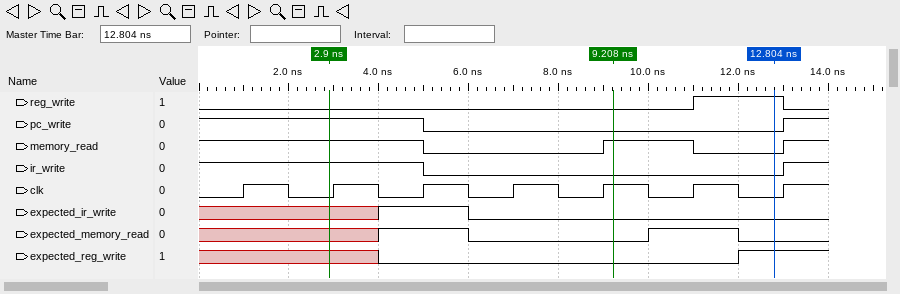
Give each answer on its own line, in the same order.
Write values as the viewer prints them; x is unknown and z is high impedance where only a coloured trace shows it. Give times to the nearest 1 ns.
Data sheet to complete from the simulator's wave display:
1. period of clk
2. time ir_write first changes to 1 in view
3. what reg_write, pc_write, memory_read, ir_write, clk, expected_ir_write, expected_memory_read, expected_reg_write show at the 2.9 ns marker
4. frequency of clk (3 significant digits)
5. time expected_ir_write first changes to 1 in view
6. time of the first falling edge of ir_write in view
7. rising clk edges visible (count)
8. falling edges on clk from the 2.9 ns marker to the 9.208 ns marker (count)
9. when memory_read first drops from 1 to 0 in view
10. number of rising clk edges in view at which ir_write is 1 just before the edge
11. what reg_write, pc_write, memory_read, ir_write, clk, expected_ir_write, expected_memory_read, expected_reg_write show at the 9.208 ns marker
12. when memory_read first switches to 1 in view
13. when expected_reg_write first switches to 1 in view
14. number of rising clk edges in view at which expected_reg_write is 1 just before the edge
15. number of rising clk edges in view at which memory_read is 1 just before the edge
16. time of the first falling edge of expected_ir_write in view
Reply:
2 ns
13 ns
reg_write=0, pc_write=1, memory_read=1, ir_write=1, clk=0, expected_ir_write=x, expected_memory_read=x, expected_reg_write=x
500 MHz
4 ns
5 ns
7
3
5 ns
3
reg_write=0, pc_write=0, memory_read=1, ir_write=0, clk=1, expected_ir_write=0, expected_memory_read=0, expected_reg_write=0
9 ns
12 ns
1
4
6 ns
